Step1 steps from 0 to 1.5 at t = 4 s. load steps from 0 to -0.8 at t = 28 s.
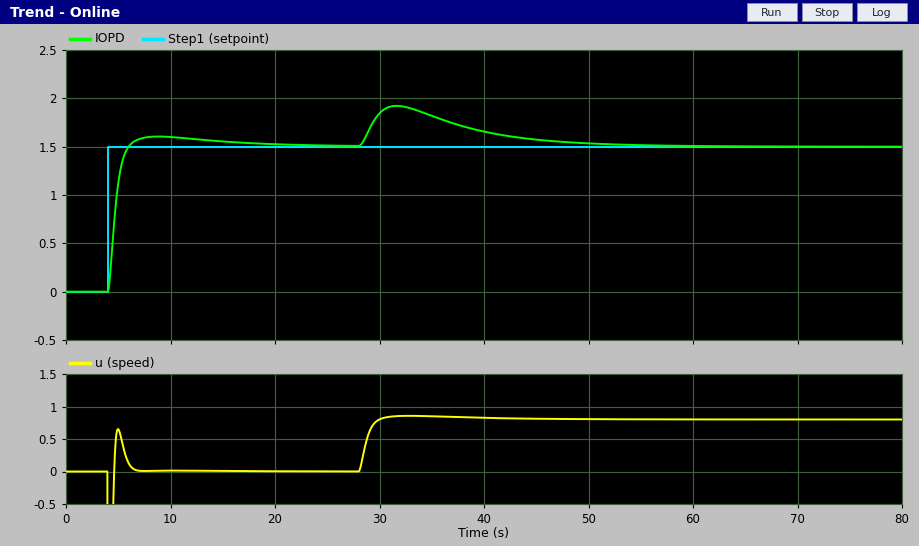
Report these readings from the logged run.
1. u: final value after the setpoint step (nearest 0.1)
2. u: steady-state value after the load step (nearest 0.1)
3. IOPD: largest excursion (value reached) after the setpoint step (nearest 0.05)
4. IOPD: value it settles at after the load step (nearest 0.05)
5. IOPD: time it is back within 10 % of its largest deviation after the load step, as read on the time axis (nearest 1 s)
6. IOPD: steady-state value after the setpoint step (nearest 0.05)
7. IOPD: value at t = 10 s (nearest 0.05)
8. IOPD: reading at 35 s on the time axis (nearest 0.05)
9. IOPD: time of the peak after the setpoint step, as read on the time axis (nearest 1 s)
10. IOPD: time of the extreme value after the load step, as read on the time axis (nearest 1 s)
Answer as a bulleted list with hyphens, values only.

- 0.0
- 0.8
- 1.60
- 1.50
- 49 s
- 1.50
- 1.60
- 1.80
- 9 s
- 32 s
